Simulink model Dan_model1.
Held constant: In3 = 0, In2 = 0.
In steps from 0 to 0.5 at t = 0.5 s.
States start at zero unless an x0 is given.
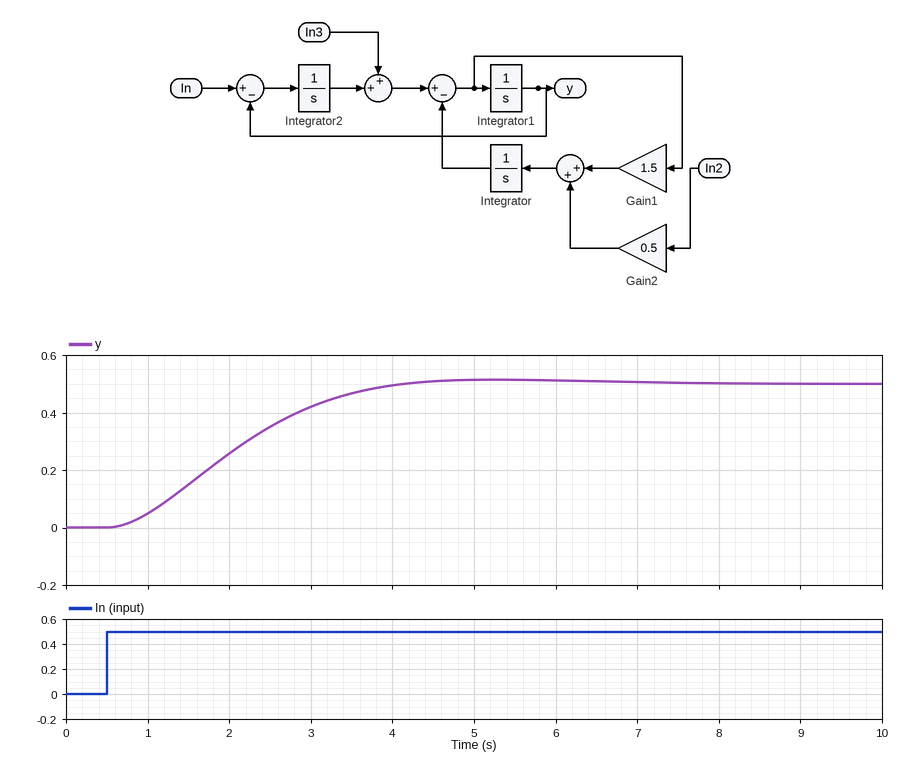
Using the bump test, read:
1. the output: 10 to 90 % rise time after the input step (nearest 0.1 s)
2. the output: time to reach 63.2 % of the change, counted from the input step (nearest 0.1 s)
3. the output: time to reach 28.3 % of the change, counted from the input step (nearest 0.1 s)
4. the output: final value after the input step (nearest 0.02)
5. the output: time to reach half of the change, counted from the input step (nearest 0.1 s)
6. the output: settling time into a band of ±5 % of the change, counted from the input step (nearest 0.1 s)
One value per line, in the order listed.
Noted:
2.3 s
1.8 s
1.0 s
0.50
1.5 s
3.1 s
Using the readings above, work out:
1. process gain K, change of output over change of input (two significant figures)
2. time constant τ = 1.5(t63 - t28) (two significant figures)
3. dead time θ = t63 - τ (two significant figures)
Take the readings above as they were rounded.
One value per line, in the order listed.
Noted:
1.0
1.2 s
0.60 s
